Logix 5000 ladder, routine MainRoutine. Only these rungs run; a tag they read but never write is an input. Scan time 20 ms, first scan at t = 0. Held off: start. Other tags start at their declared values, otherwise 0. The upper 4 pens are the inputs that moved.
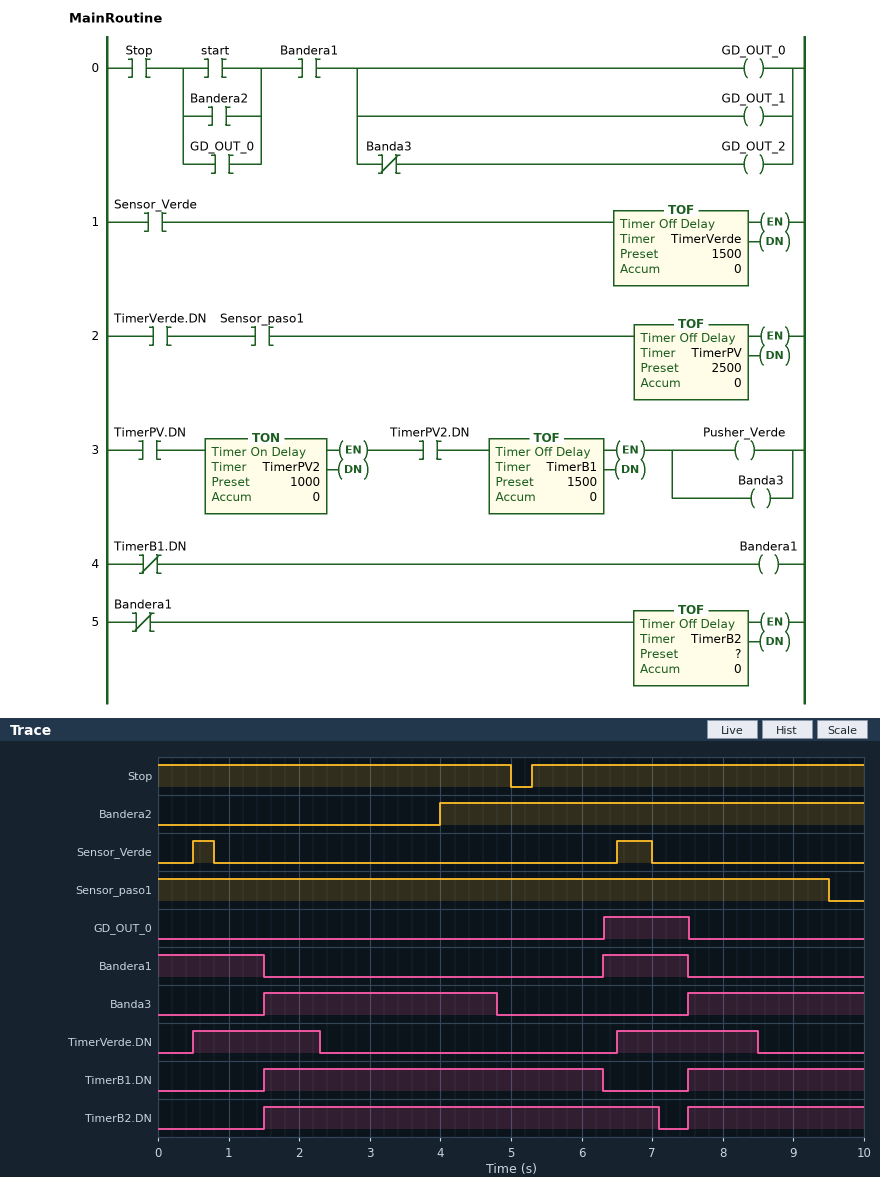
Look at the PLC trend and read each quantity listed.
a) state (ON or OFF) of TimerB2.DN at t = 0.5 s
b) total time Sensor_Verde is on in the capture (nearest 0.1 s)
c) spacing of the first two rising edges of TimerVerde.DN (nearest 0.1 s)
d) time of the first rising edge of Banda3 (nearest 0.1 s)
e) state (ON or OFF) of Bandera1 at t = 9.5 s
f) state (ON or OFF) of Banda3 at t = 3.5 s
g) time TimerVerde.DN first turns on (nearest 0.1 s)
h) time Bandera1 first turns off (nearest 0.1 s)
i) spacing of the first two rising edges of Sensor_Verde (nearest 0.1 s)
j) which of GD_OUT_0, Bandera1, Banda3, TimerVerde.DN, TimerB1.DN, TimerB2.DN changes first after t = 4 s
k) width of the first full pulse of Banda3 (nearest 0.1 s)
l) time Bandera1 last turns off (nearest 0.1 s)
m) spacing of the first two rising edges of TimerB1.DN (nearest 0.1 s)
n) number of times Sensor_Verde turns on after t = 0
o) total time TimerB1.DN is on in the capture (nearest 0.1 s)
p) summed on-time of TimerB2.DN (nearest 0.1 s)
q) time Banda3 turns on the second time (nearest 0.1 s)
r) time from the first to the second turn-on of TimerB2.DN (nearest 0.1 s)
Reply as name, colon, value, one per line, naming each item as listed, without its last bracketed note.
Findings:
state (ON or OFF) of TimerB2.DN at t = 0.5 s: OFF
total time Sensor_Verde is on in the capture: 0.8 s
spacing of the first two rising edges of TimerVerde.DN: 6.0 s
time of the first rising edge of Banda3: 1.5 s
state (ON or OFF) of Bandera1 at t = 9.5 s: OFF
state (ON or OFF) of Banda3 at t = 3.5 s: ON
time TimerVerde.DN first turns on: 0.5 s
time Bandera1 first turns off: 1.5 s
spacing of the first two rising edges of Sensor_Verde: 6.0 s
which of GD_OUT_0, Bandera1, Banda3, TimerVerde.DN, TimerB1.DN, TimerB2.DN changes first after t = 4 s: Banda3
width of the first full pulse of Banda3: 3.3 s
time Bandera1 last turns off: 7.5 s
spacing of the first two rising edges of TimerB1.DN: 6.0 s
number of times Sensor_Verde turns on after t = 0: 2
total time TimerB1.DN is on in the capture: 7.3 s
summed on-time of TimerB2.DN: 8.1 s
time Banda3 turns on the second time: 7.5 s
time from the first to the second turn-on of TimerB2.DN: 6.0 s
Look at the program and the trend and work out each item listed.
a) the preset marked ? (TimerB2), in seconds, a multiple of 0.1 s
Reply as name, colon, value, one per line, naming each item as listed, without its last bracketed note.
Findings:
the preset marked ? (TimerB2), in seconds, a multiple of 0.1 s: 0.8 s
